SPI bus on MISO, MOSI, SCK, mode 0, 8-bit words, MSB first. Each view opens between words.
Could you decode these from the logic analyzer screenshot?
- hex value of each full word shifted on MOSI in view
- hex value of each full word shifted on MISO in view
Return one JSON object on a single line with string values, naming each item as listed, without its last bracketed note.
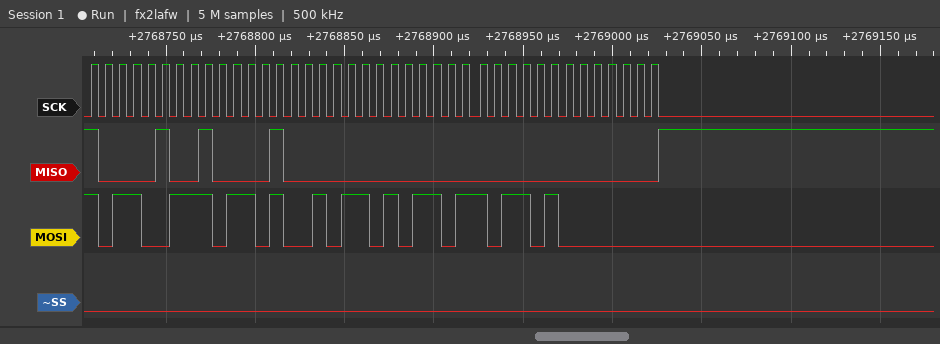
{"hex value of each full word shifted on MOSI in view": "B3, B4, B5, B6, 80", "hex value of each full word shifted on MISO in view": "84, 84, 00, 00, 00"}
